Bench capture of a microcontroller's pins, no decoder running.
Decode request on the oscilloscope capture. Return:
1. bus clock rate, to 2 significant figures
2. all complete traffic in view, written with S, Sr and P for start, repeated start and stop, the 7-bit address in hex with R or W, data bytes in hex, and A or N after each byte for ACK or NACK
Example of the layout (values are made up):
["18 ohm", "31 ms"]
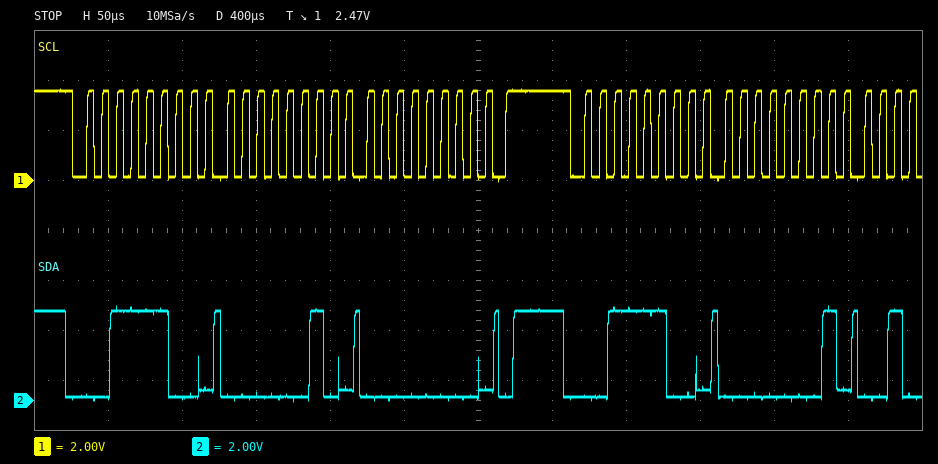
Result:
["100 kHz", "S 1EW A 02 A 00 A P S 1EW A 01 A"]
